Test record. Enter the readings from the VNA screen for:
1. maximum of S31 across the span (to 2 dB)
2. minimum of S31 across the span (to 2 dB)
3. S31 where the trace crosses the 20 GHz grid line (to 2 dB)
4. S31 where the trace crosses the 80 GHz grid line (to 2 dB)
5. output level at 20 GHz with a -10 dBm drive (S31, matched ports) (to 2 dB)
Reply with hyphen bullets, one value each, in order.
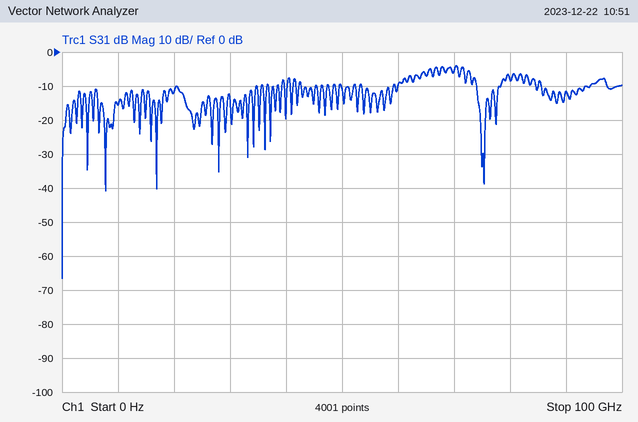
- -4 dB
- -66 dB
- -12 dB
- -8 dB
- -22 dBm
